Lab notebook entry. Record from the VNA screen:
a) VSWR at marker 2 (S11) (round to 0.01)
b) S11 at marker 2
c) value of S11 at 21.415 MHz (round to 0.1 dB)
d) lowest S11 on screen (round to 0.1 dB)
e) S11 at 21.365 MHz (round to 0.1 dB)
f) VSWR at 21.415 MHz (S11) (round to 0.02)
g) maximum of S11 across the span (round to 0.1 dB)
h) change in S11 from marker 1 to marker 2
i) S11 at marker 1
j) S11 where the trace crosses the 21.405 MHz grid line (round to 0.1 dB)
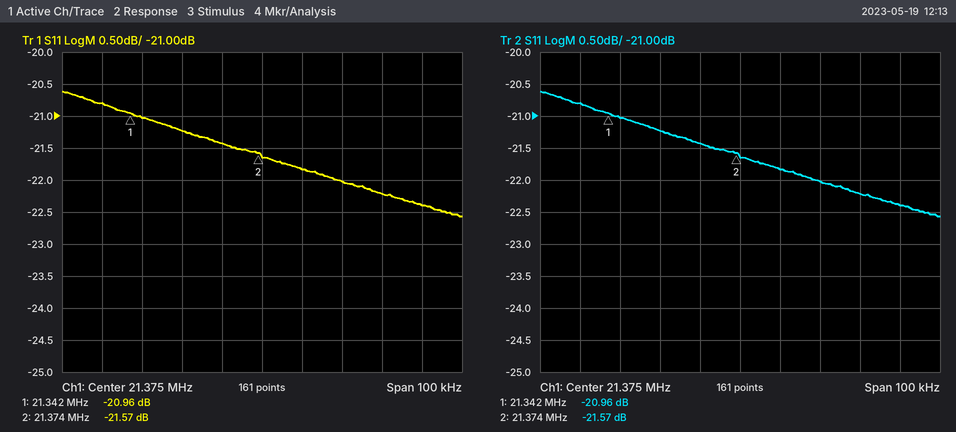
1.18
-21.57 dB
-22.4 dB
-22.6 dB
-21.4 dB
1.16
-20.6 dB
-0.61 dB
-20.96 dB
-22.2 dB
